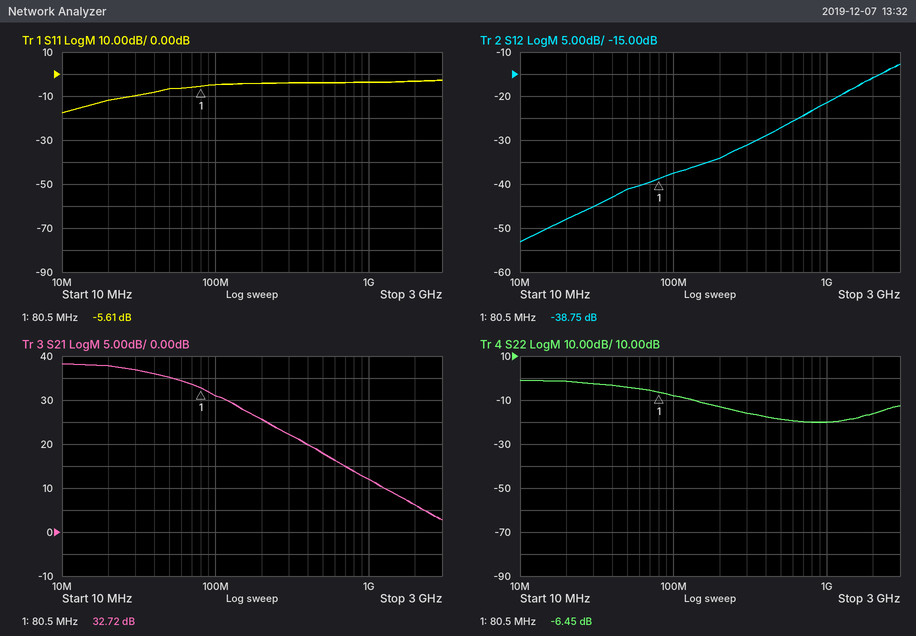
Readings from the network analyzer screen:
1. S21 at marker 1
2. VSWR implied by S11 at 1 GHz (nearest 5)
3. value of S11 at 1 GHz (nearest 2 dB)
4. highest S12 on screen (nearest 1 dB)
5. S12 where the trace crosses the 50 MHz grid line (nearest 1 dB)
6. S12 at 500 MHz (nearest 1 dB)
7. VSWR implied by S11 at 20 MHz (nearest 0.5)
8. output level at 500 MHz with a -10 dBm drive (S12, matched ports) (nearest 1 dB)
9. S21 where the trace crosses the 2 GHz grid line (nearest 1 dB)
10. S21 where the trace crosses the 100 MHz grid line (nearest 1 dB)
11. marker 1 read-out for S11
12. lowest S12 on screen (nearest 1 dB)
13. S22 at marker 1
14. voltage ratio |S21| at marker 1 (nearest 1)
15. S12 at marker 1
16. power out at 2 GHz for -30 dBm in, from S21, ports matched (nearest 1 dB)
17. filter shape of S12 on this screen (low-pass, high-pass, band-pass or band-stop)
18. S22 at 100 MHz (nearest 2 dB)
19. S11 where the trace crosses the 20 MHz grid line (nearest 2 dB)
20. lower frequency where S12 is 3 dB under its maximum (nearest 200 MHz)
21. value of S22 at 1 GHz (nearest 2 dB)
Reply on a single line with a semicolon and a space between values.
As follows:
32.72 dB; 5; -4 dB; -13 dB; -41 dB; -27 dB; 1.5; -37 dBm; 6 dB; 31 dB; -5.61 dB; -53 dB; -6.45 dB; 43; -38.75 dB; -24 dBm; high-pass; -8 dB; -12 dB; 2.0 GHz; -20 dB
